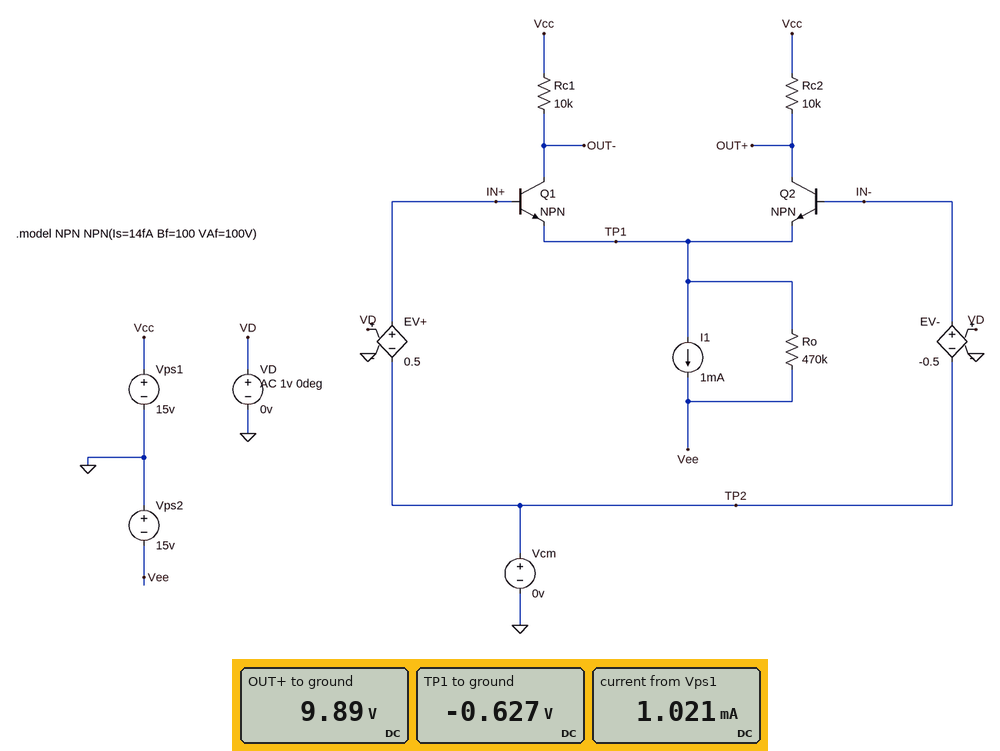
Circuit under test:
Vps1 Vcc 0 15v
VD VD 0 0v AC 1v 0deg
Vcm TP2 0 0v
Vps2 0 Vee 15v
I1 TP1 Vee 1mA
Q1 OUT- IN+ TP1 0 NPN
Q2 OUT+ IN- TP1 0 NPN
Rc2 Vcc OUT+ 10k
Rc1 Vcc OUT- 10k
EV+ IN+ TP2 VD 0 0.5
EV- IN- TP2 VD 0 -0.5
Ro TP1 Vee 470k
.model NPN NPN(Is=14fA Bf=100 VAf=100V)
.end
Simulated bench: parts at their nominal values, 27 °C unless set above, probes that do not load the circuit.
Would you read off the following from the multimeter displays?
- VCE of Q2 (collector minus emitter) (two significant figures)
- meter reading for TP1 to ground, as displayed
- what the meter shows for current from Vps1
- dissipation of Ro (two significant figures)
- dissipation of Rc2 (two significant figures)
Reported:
11 V
-0.627 V
1.021 mA
440 µW
2.6 mW
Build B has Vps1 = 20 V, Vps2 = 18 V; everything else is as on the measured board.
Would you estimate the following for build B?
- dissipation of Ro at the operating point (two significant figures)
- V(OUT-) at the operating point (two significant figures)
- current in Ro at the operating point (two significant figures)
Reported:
640 µW
15 V
37 µA
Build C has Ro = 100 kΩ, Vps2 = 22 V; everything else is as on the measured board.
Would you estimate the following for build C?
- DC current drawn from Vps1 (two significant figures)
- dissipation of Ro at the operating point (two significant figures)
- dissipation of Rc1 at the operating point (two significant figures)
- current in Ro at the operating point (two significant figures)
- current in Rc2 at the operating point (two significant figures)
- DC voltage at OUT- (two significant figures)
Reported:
1.2 mA
4.6 mW
3.6 mW
210 µA
600 µA
9.0 V
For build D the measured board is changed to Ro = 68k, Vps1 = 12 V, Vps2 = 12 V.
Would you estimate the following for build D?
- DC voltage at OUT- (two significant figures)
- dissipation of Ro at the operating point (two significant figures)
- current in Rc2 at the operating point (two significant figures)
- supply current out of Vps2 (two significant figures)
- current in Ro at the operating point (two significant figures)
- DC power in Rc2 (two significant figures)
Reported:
6.2 V
1.9 mW
580 µA
1.2 mA
170 µA
3.3 mW
